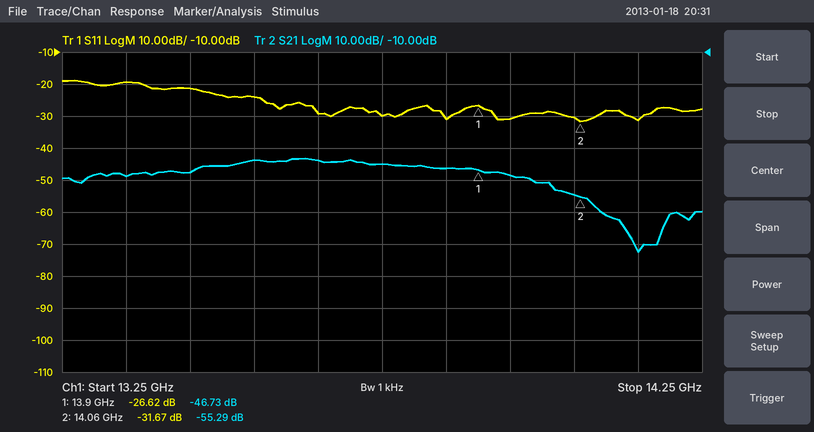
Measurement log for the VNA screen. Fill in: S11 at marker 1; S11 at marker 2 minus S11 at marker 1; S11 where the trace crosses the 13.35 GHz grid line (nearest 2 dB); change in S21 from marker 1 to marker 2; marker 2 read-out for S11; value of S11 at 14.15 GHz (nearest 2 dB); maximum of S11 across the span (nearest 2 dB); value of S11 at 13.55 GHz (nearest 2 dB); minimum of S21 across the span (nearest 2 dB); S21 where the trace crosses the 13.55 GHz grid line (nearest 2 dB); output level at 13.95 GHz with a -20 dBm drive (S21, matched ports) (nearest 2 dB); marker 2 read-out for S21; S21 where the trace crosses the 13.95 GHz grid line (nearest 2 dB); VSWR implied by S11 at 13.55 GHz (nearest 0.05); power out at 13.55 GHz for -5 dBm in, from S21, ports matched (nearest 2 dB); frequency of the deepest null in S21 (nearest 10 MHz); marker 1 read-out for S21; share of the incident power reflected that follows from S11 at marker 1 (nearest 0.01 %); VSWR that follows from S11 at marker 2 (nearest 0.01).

-26.62 dB
-5.05 dB
-20 dB
-8.56 dB
-31.67 dB
-32 dB
-18 dB
-24 dB
-72 dB
-44 dB
-68 dBm
-55.29 dB
-48 dB
1.15
-48 dBm
14.15 GHz
-46.73 dB
0.22 %
1.05
